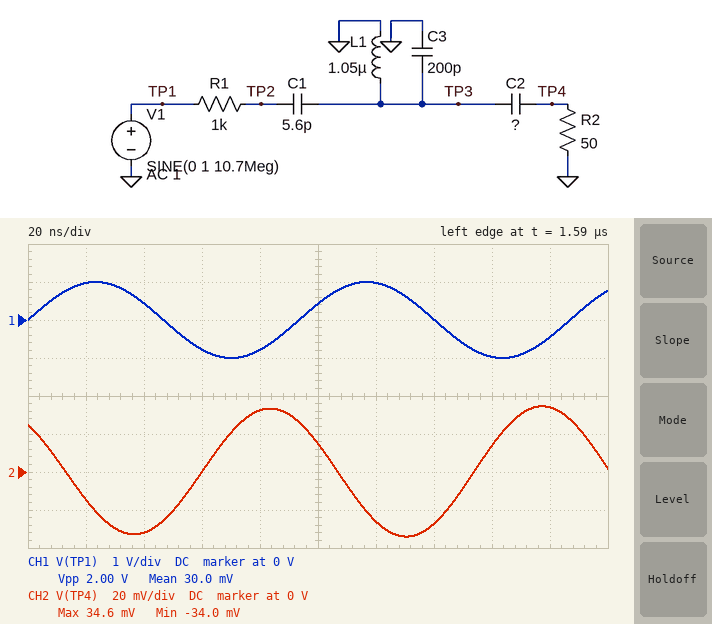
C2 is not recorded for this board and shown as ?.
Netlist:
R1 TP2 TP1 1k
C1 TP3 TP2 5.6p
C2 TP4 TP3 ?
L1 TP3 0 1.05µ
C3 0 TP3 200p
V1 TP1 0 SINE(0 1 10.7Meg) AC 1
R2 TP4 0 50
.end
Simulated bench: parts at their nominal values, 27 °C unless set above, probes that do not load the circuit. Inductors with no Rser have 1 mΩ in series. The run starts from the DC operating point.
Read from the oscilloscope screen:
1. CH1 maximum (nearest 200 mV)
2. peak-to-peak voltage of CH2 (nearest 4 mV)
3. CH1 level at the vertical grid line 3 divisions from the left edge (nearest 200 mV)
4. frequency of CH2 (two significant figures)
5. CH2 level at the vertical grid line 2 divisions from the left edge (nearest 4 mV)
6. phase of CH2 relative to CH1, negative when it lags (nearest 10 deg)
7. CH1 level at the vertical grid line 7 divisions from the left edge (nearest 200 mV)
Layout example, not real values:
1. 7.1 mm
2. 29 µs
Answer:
1. 1.0 V
2. 68 mV
3. -800 mV
4. 11 MHz
5. -32 mV
6. 130 deg
7. 0 V
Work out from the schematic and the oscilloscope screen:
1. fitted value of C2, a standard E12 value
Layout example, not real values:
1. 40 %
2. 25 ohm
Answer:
1. 10 pF
